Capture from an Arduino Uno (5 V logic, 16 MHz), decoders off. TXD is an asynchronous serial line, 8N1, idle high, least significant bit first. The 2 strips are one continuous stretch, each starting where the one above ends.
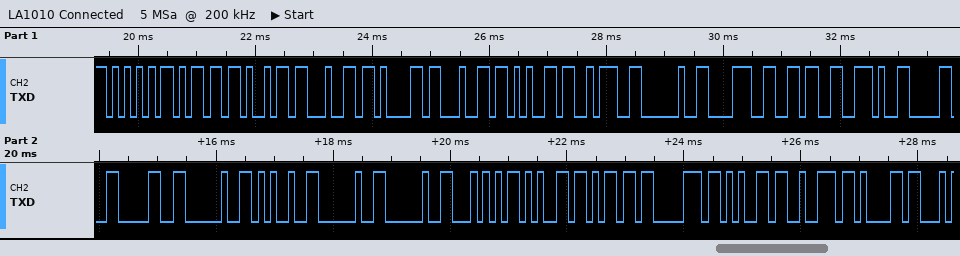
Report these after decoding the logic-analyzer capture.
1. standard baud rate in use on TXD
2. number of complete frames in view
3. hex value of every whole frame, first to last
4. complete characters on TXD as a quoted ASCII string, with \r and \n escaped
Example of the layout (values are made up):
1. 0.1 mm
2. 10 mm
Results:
1. 9600 baud
2. 25
3. 55 6D 69 64 61 64 65 3A 20 38 36 2E 30 30 20 25 20 20 54 65 6D 70 65 72 61
4. "Umidade: 86.00 %  Tempera"
